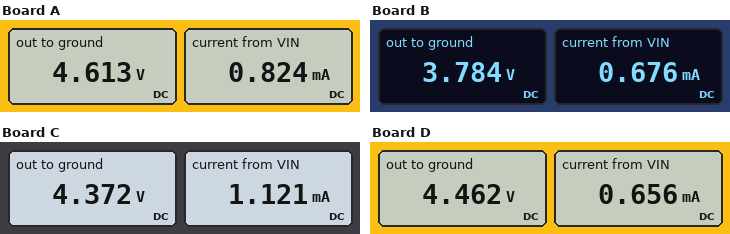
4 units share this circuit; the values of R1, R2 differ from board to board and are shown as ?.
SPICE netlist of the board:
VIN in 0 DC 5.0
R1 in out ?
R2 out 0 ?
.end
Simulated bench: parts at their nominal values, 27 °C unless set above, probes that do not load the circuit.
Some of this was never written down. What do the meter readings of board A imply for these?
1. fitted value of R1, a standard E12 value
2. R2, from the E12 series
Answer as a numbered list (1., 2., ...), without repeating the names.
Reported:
1. 470 Ω
2. 5.6 kΩ
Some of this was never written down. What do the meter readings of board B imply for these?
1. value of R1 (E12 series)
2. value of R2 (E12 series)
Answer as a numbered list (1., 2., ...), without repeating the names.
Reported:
1. 1.8 kΩ
2. 5.6 kΩ
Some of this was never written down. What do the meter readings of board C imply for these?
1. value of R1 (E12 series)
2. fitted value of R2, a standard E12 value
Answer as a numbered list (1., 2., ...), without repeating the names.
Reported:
1. 560 Ω
2. 3.9 kΩ
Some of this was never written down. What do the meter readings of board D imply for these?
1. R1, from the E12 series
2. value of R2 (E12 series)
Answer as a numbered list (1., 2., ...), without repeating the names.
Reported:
1. 820 Ω
2. 6.8 kΩ
